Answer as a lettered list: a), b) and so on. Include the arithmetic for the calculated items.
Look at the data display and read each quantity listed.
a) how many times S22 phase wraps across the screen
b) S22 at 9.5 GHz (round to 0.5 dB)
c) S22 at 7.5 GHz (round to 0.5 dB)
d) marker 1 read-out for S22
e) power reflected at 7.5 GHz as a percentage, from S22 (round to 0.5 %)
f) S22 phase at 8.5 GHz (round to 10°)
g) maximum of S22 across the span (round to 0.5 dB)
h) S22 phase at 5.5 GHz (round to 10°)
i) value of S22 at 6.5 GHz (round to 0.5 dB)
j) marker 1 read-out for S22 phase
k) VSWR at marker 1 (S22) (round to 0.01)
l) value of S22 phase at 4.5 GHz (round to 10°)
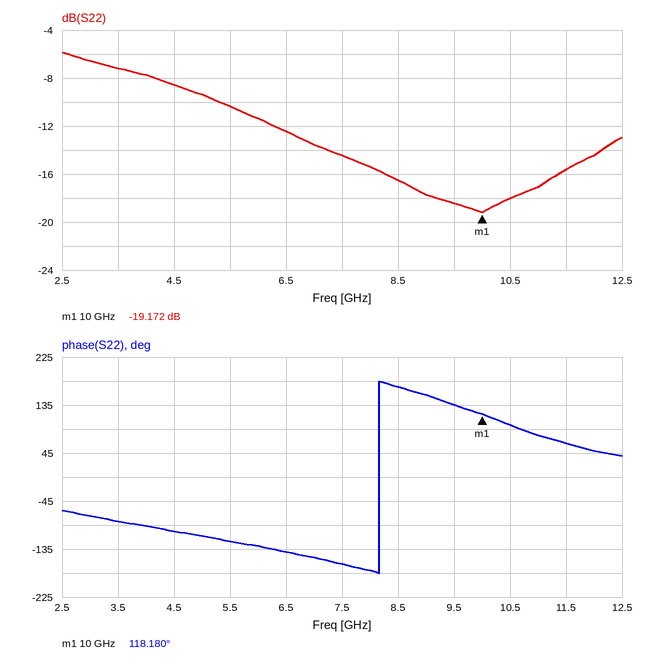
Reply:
a) 1
b) -18.5 dB
c) -14.5 dB
d) -19.172 dB
e) 10^(-14.5/10) ≈ 3.5 %
f) 170°
g) -6.0 dB
h) -120°
i) -12.5 dB
j) 118.180°
k) (1 + 0.1100)/(1 − 0.1100) ≈ 1.25
l) -100°
